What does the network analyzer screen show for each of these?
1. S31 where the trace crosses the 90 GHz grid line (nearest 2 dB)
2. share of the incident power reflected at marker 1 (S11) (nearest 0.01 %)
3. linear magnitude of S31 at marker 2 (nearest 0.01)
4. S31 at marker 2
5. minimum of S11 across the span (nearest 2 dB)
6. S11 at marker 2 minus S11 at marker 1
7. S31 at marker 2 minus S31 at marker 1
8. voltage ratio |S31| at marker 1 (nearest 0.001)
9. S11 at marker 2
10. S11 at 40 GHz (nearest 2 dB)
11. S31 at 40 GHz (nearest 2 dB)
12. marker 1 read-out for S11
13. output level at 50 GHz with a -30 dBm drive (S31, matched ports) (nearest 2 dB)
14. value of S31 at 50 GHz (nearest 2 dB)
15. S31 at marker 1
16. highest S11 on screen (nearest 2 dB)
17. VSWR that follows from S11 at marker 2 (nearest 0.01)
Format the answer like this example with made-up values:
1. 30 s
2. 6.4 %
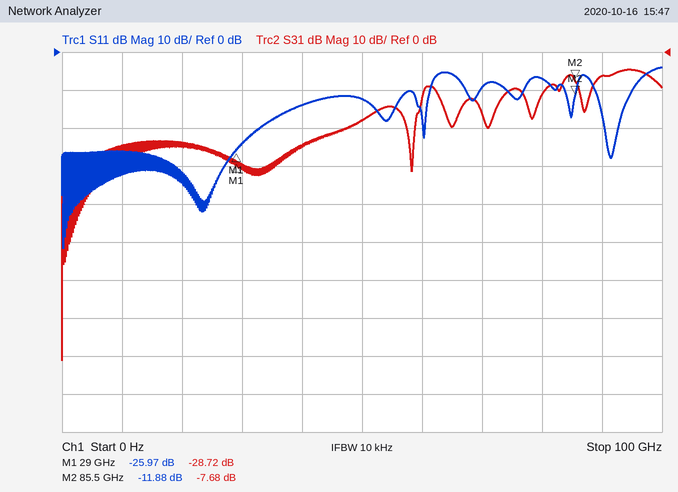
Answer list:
1. -6 dB
2. 0.25 %
3. 0.41
4. -7.68 dB
5. -52 dB
6. 14.09 dB
7. 21.04 dB
8. 0.037
9. -11.88 dB
10. -14 dB
11. -24 dB
12. -25.97 dB
13. -48 dBm
14. -18 dB
15. -28.72 dB
16. -4 dB
17. 1.68
